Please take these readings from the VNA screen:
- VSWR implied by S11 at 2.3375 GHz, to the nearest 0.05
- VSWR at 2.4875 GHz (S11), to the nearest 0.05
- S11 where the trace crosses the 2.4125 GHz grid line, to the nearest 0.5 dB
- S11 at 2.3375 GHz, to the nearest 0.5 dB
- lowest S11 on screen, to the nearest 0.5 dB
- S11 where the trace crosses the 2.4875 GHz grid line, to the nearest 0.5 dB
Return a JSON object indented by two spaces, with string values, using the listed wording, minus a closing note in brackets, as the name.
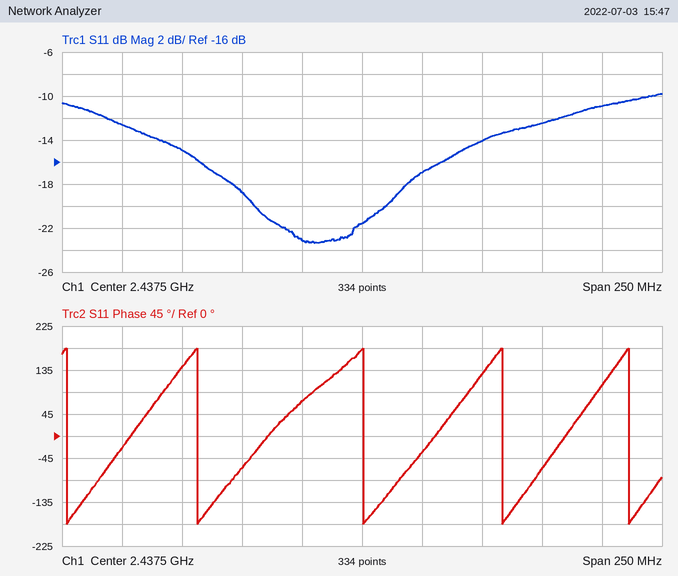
{
  "VSWR implied by S11 at 2.3375 GHz, to the nearest 0.05": "1.60",
  "VSWR at 2.4875 GHz (S11), to the nearest 0.05": "1.50",
  "S11 where the trace crosses the 2.4125 GHz grid line, to the nearest 0.5 dB": "-23.0 dB",
  "S11 at 2.3375 GHz, to the nearest 0.5 dB": "-12.5 dB",
  "lowest S11 on screen, to the nearest 0.5 dB": "-23.5 dB",
  "S11 where the trace crosses the 2.4875 GHz grid line, to the nearest 0.5 dB": "-14.0 dB"
}
